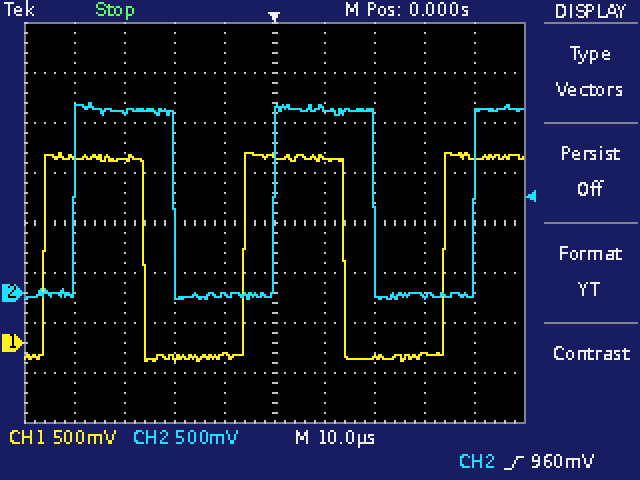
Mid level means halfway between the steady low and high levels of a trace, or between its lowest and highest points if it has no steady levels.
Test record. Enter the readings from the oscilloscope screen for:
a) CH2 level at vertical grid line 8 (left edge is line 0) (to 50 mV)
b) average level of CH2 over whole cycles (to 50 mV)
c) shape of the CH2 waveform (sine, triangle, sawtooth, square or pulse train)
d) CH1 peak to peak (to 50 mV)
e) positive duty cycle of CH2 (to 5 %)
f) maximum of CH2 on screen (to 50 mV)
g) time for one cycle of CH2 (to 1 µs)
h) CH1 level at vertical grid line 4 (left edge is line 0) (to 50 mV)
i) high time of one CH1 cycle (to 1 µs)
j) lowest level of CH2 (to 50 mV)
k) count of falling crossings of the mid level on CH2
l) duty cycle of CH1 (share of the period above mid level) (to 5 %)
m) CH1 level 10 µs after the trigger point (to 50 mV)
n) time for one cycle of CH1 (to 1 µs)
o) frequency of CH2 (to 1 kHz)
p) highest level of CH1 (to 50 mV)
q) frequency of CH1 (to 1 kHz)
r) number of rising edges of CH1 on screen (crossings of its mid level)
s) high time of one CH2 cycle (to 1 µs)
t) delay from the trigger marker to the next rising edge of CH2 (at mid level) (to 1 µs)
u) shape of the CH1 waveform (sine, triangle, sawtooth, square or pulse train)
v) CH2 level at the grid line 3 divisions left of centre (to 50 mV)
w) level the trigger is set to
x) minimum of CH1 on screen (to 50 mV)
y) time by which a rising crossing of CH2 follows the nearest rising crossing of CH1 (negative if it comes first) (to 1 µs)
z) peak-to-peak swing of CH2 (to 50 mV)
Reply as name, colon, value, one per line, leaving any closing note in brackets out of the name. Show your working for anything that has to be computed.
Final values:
CH2 level at vertical grid line 8 (left edge is line 0): -50 mV
average level of CH2 over whole cycles: -50 mV + 0.5 × (1.90 V − (-50 mV)) ≈ 925 mV, so 900 mV to the nearest 50 mV
shape of the CH2 waveform: square
CH1 peak to peak: 1.90 V − (-200 mV) = 2.10 V
positive duty cycle of CH2: 20 µs / 40 µs ≈ 50 %
maximum of CH2 on screen: 1.90 V
time for one cycle of CH2: 40 µs
CH1 level at vertical grid line 4 (left edge is line 0): -100 mV
high time of one CH1 cycle: 20 µs
lowest level of CH2: -50 mV
count of falling crossings of the mid level on CH2: 2
duty cycle of CH1 (share of the period above mid level): 20 µs / 40 µs ≈ 50 %
CH1 level 10 µs after the trigger point: 1.85 V
time for one cycle of CH1: 40 µs
frequency of CH2: 1 / 40 µs ≈ 25 kHz
highest level of CH1: 1.90 V
frequency of CH1: 1 / 40 µs ≈ 25 kHz
number of rising edges of CH1 on screen: 3
high time of one CH2 cycle: 20 µs
delay from the trigger marker to the next rising edge of CH2 (at mid level): 40 µs
shape of the CH1 waveform: square
CH2 level at the grid line 3 divisions left of centre: 1.80 V
level the trigger is set to: 960 mV
minimum of CH1 on screen: -200 mV
time by which a rising crossing of CH2 follows the nearest rising crossing of CH1 (negative if it comes first): +6 µs
peak-to-peak swing of CH2: 1.90 V − (-50 mV) = 1.95 V
